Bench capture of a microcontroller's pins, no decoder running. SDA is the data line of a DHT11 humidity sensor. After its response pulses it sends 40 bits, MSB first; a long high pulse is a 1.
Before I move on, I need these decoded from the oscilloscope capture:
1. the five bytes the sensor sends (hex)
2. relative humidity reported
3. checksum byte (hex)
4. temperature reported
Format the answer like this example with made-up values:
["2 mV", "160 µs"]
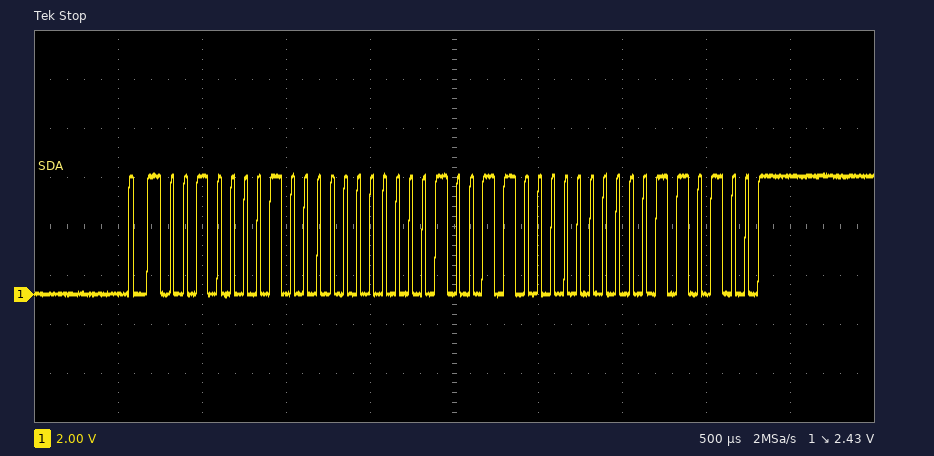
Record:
["21 00 13 00 34", "33 %", "0x34", "19.0 °C"]
